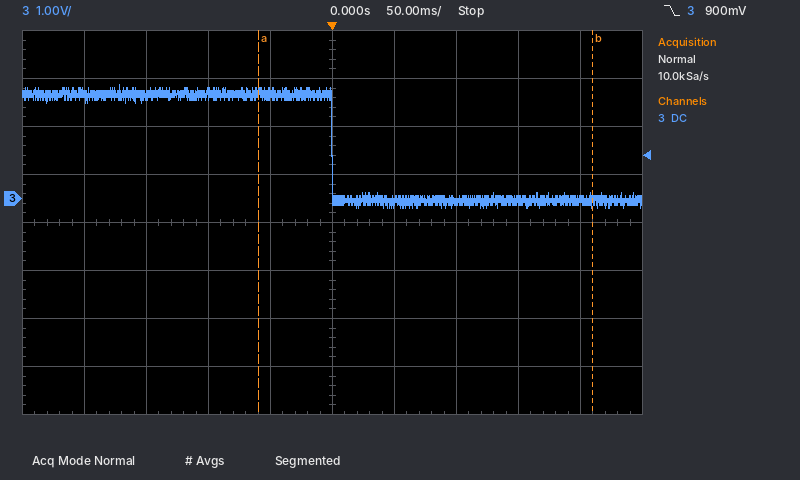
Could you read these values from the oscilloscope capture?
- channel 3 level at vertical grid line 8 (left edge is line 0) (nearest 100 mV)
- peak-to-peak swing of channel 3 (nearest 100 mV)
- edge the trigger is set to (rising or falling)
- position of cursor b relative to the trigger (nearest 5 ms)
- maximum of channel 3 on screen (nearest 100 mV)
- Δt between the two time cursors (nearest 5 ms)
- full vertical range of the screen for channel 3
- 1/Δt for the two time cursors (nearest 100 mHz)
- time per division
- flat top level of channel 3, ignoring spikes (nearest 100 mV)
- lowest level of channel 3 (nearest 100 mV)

0.0 V
2.6 V
falling
+210 ms
2.4 V
270 ms
8 V
3.7 Hz
50 ms
2.2 V
-200 mV
